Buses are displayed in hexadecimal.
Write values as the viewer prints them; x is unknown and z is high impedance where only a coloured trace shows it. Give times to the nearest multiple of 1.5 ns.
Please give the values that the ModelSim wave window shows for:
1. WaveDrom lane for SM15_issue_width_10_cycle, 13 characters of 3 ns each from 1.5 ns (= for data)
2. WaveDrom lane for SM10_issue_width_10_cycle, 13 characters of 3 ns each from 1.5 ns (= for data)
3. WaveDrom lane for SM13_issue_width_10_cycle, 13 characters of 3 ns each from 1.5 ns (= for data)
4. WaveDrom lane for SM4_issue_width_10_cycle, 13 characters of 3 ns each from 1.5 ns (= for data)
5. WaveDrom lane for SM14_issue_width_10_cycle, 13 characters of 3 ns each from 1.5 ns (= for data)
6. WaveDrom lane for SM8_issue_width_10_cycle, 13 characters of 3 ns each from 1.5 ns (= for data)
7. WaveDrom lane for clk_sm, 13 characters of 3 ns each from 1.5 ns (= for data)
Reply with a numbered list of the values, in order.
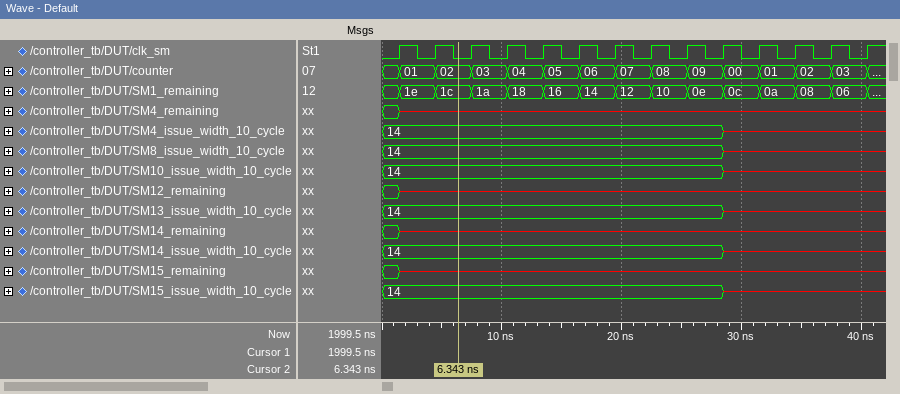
1. {name: 'SM15_issue_width_10_cycle', wave: '=........x...', data: '14'}
2. {name: 'SM10_issue_width_10_cycle', wave: '=........x...', data: '14'}
3. {name: 'SM13_issue_width_10_cycle', wave: '=........x...', data: '14'}
4. {name: 'SM4_issue_width_10_cycle', wave: '=........x...', data: '14'}
5. {name: 'SM14_issue_width_10_cycle', wave: '=........x...', data: '14'}
6. {name: 'SM8_issue_width_10_cycle', wave: '=........x...', data: '14'}
7. {name: 'clk_sm', wave: 'p............'}
